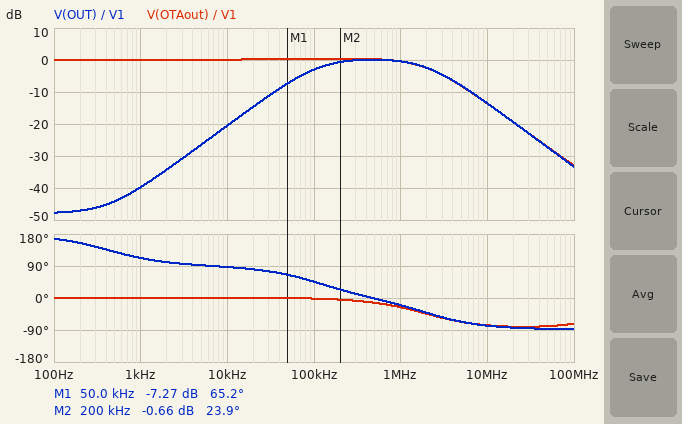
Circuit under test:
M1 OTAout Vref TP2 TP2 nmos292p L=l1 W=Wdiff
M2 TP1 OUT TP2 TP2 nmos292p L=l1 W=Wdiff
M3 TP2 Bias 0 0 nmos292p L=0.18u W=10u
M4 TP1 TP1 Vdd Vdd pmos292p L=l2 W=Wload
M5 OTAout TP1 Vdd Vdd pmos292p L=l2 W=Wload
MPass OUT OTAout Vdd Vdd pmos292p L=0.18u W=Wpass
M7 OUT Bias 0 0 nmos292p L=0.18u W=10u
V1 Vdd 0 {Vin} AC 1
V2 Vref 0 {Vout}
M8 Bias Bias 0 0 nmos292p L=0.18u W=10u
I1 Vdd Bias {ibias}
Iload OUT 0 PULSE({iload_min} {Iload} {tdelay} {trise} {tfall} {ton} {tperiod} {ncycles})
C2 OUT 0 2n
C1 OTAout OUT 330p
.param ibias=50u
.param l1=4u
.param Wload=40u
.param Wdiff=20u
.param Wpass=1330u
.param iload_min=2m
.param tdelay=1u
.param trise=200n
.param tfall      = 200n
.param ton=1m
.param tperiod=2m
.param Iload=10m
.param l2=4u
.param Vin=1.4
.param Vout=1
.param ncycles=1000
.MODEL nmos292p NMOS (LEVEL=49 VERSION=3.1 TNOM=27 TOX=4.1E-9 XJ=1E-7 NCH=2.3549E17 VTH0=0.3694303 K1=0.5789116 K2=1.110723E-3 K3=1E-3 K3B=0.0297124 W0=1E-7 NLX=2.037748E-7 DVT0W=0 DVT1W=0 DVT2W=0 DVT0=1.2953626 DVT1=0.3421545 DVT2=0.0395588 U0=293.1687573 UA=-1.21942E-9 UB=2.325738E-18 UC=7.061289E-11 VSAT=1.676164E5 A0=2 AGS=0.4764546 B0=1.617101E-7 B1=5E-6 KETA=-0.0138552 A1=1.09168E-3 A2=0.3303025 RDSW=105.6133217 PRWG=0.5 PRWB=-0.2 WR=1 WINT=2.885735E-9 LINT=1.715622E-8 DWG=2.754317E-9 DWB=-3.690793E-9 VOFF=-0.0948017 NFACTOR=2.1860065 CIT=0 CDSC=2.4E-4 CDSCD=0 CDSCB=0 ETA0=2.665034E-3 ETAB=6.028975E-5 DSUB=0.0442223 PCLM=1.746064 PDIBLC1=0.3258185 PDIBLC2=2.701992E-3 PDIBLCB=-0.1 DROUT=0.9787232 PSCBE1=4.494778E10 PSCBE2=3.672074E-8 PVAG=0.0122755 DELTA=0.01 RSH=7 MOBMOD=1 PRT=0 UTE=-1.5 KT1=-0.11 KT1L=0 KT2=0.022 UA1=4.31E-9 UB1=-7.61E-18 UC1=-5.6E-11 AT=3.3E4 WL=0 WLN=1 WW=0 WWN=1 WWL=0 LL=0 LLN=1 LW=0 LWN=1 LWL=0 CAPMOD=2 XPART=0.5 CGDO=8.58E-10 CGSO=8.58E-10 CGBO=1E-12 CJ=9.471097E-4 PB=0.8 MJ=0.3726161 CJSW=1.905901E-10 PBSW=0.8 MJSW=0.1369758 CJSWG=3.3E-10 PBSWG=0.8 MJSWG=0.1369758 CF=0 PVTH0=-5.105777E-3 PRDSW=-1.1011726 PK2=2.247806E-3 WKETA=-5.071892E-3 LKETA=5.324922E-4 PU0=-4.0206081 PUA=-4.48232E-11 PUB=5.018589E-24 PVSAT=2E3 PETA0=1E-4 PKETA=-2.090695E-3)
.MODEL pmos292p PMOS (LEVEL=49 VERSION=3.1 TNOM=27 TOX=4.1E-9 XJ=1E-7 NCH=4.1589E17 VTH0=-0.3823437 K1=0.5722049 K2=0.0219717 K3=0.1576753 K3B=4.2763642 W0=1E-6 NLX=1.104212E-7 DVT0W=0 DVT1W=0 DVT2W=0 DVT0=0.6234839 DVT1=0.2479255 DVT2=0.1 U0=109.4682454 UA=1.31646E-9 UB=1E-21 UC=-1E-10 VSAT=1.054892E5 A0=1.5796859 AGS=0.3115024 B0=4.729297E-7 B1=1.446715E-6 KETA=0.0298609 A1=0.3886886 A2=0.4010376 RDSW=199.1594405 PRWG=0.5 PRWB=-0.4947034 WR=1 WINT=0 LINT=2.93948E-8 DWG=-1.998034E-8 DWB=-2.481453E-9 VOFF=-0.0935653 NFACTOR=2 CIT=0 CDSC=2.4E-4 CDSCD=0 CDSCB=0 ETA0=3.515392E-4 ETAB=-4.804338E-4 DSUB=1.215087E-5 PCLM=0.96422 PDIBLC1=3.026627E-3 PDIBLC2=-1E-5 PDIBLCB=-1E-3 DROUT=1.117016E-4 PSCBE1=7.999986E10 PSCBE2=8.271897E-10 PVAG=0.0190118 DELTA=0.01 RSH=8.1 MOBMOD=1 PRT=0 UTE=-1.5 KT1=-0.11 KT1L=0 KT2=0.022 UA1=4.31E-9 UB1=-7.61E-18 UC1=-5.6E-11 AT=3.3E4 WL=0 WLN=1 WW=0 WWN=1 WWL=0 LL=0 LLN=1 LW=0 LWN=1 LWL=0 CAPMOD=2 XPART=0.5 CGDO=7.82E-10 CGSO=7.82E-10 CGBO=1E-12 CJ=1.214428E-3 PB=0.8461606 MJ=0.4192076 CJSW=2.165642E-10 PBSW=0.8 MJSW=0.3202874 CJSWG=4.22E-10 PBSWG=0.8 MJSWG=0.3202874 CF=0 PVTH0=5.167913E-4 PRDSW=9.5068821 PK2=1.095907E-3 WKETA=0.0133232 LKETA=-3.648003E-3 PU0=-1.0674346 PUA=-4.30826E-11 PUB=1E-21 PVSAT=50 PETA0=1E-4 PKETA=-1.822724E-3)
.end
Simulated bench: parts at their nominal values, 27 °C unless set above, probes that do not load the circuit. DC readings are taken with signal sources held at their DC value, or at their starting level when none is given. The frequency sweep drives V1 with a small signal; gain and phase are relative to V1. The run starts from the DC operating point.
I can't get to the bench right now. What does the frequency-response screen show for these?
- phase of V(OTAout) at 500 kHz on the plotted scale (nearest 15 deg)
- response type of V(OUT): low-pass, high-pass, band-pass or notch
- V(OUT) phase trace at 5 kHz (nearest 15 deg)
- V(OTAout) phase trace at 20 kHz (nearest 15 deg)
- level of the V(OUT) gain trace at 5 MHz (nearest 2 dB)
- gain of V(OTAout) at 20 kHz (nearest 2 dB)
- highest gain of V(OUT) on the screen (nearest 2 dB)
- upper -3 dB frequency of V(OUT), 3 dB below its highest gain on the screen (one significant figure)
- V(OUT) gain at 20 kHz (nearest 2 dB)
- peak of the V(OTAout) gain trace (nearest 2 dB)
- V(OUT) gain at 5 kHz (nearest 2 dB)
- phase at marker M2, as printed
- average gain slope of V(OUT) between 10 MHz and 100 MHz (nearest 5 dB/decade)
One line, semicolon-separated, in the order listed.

-15 deg; band-pass; 90 deg; 0 deg; -8 dB; 0 dB; 0 dB; 2 MHz; -14 dB; 0 dB; -26 dB; 23.9 deg; -20 dB/decade
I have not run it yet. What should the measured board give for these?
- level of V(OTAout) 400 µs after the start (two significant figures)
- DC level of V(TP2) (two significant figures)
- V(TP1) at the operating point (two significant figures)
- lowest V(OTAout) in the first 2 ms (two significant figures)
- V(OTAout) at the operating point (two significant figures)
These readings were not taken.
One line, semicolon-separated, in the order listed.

640 mV; 410 mV; 720 mV; 640 mV; 840 mV
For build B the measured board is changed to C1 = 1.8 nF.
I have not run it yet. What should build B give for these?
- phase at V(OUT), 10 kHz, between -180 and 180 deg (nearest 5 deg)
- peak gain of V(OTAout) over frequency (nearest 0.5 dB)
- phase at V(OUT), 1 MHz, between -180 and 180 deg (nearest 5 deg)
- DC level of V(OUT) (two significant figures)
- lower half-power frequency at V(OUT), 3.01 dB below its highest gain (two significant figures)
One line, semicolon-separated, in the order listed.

65 deg; 0 dB; -25 deg; 1.0 V; 19 kHz
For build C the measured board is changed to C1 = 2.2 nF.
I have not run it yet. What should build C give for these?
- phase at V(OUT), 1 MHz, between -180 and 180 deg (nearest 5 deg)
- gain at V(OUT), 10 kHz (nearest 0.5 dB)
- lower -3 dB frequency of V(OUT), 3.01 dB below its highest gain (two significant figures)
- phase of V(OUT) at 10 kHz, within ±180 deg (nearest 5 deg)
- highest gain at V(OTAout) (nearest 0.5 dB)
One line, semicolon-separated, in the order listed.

-25 deg; -5.5 dB; 16 kHz; 60 deg; 0 dB
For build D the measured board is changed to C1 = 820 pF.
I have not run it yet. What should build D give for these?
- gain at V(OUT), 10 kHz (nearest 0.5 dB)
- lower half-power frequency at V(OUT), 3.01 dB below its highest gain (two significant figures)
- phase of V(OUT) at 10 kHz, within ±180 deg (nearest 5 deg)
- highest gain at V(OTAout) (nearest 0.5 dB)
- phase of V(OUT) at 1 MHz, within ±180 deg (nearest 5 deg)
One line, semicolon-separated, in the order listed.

-13.0 dB; 42 kHz; 80 deg; 0 dB; -25 deg
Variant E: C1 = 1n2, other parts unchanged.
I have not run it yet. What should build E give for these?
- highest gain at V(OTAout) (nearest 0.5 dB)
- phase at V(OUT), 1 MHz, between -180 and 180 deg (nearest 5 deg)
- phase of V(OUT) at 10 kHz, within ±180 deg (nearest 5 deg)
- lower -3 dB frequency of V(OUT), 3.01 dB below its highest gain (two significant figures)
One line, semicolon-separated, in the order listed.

0 dB; -25 deg; 70 deg; 29 kHz
